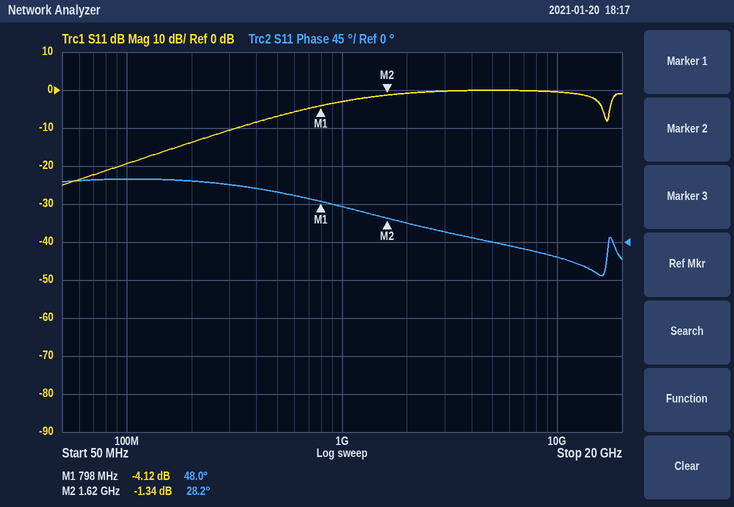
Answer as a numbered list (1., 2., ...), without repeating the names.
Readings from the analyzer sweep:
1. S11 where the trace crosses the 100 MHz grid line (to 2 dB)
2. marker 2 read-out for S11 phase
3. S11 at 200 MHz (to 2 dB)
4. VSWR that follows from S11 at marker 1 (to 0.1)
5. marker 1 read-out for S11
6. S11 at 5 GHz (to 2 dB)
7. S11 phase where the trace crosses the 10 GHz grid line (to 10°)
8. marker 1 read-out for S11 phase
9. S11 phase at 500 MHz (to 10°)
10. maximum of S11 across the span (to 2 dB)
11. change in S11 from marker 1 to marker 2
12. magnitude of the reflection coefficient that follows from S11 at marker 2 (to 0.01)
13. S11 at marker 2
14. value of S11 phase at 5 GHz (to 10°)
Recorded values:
1. -20 dB
2. 28.2°
3. -14 dB
4. 4.3
5. -4.12 dB
6. 0 dB
7. -20°
8. 48.0°
9. 60°
10. 0 dB
11. 2.78 dB
12. 0.86
13. -1.34 dB
14. 0°
